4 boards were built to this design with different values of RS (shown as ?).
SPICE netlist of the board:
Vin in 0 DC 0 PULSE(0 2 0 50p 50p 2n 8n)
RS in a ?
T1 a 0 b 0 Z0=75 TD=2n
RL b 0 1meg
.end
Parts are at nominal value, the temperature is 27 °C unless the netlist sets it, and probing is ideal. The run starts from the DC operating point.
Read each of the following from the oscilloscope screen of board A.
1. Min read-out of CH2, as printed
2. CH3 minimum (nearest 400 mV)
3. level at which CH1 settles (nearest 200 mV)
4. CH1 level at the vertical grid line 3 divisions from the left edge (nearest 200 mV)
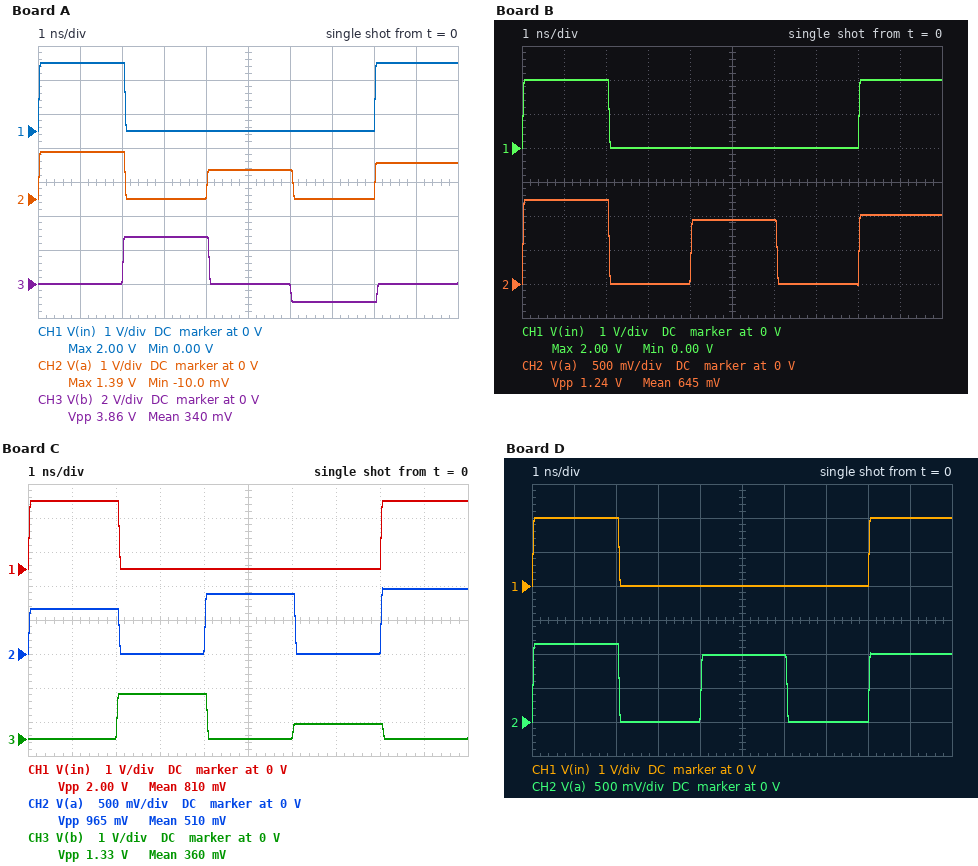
-10.0 mV
-1.2 V
2.0 V
0 V
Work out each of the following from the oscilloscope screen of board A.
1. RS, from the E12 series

33 Ω
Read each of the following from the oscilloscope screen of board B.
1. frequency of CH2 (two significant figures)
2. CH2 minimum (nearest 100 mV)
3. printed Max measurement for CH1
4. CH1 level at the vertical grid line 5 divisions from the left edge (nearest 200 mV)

250 MHz
0 V
2.00 V
0 V
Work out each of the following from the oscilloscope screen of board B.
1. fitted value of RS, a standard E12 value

47 Ω
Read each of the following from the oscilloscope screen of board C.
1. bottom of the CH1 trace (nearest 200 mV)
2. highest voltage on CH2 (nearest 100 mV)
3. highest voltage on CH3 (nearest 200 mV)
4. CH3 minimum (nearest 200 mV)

0 V
1.0 V
1.4 V
0 V
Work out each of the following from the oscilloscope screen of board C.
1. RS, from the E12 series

150 Ω
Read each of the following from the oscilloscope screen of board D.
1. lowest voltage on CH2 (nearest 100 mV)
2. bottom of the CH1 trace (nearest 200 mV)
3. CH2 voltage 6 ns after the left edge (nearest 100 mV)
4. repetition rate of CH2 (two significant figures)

0 V
0 V
1.0 V
250 MHz
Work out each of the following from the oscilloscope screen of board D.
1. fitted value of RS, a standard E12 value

56 Ω
